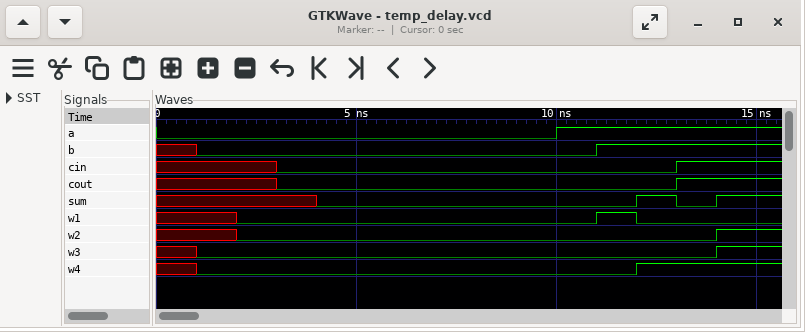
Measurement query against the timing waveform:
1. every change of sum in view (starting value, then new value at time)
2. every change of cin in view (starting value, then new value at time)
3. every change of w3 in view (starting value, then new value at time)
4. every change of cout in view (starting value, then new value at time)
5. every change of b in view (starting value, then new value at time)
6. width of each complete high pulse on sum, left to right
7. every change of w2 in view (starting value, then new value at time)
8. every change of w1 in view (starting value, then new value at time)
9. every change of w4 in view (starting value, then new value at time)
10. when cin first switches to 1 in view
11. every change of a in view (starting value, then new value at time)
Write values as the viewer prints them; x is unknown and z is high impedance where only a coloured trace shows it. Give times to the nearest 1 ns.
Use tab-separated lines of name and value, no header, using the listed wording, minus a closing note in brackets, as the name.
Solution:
every change of sum in view	x, 0 at 4 ns, 1 at 12 ns, 0 at 13 ns, 1 at 14 ns
every change of cin in view	x, 0 at 3 ns, 1 at 13 ns
every change of w3 in view	x, 0 at 1 ns, 1 at 14 ns
every change of cout in view	x, 0 at 3 ns, 1 at 13 ns
every change of b in view	x, 0 at 1 ns, 1 at 11 ns
width of each complete high pulse on sum, left to right	1 ns
every change of w2 in view	x, 0 at 2 ns, 1 at 14 ns
every change of w1 in view	x, 0 at 2 ns, 1 at 11 ns, 0 at 12 ns
every change of w4 in view	x, 0 at 1 ns, 1 at 12 ns
when cin first switches to 1 in view	13 ns
every change of a in view	0, 1 at 10 ns
